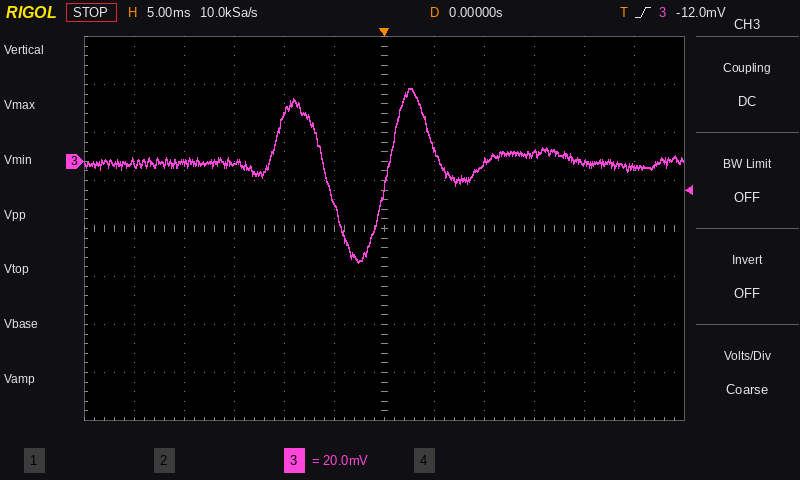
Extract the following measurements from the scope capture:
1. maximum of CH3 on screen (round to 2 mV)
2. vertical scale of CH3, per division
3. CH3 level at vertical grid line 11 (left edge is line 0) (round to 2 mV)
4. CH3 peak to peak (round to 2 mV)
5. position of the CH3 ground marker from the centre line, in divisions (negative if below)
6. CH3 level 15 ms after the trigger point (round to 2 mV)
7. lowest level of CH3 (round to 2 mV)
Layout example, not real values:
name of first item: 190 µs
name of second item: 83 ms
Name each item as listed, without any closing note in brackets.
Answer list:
maximum of CH3 on screen: 30 mV
vertical scale of CH3, per division: 20 mV
CH3 level at vertical grid line 11 (left edge is line 0): -2 mV
CH3 peak to peak: 72 mV
position of the CH3 ground marker from the centre line, in divisions: +1.4 div
CH3 level 15 ms after the trigger point: 4 mV
lowest level of CH3: -42 mV
